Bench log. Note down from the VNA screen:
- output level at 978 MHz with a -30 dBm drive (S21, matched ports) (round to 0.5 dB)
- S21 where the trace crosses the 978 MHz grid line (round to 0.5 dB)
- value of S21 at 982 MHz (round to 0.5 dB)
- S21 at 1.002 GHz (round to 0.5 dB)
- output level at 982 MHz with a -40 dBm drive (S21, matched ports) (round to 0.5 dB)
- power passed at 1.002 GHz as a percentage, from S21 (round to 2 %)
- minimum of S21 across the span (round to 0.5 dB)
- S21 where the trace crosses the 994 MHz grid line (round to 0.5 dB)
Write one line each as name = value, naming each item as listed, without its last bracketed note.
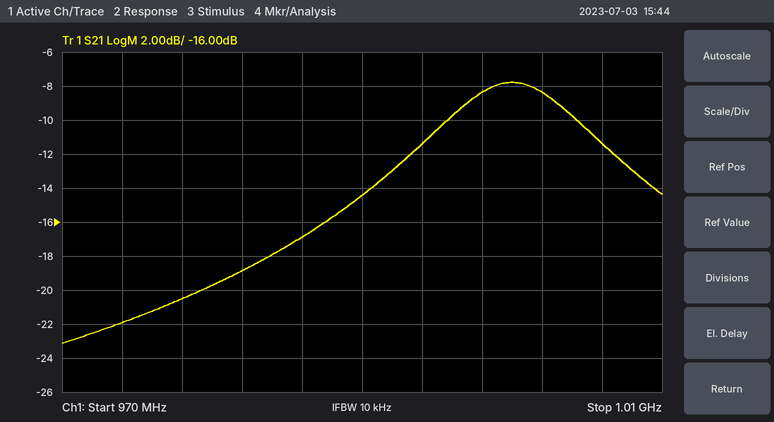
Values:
output level at 978 MHz with a -30 dBm drive (S21, matched ports) = -50.5 dBm
S21 where the trace crosses the 978 MHz grid line = -20.5 dB
value of S21 at 982 MHz = -19.0 dB
S21 at 1.002 GHz = -8.5 dB
output level at 982 MHz with a -40 dBm drive (S21, matched ports) = -59.0 dBm
power passed at 1.002 GHz as a percentage, from S21 = 14 %
minimum of S21 across the span = -23.0 dB
S21 where the trace crosses the 994 MHz grid line = -11.5 dB
